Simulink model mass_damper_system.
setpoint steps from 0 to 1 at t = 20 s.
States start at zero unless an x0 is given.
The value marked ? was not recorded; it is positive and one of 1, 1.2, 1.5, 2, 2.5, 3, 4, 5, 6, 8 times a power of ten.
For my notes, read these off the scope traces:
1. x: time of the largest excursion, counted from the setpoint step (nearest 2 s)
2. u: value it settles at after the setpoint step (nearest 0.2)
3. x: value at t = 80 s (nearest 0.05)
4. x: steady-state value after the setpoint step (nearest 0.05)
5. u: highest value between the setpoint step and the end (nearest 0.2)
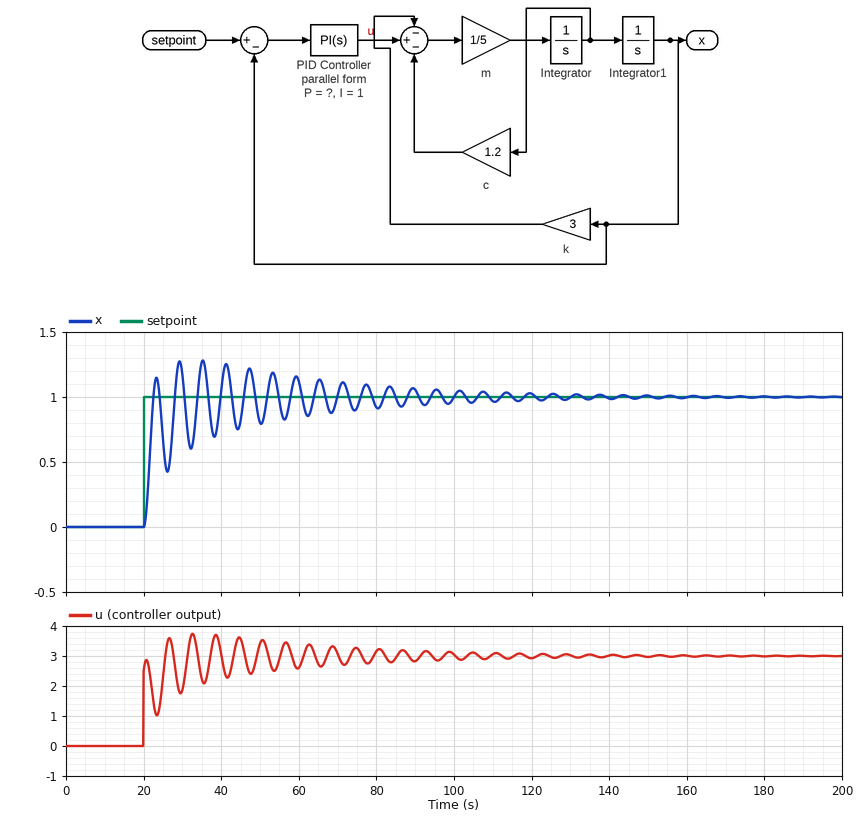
16 s
3.0
0.90
1.00
3.8
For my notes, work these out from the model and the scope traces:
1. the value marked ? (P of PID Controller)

2.5
